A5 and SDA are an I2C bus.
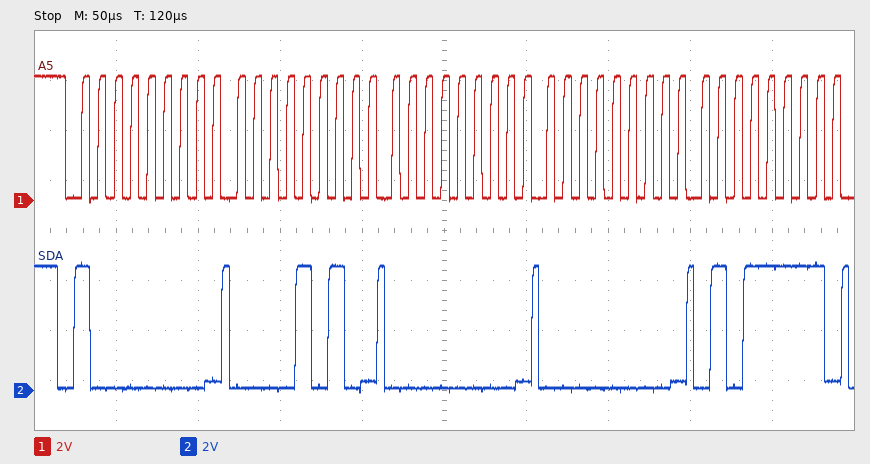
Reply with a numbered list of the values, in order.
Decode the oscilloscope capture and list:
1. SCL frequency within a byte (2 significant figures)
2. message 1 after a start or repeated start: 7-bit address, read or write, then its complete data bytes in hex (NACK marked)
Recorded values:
1. 100 kHz
2. 0x40 write: 0A 00 00 5F
